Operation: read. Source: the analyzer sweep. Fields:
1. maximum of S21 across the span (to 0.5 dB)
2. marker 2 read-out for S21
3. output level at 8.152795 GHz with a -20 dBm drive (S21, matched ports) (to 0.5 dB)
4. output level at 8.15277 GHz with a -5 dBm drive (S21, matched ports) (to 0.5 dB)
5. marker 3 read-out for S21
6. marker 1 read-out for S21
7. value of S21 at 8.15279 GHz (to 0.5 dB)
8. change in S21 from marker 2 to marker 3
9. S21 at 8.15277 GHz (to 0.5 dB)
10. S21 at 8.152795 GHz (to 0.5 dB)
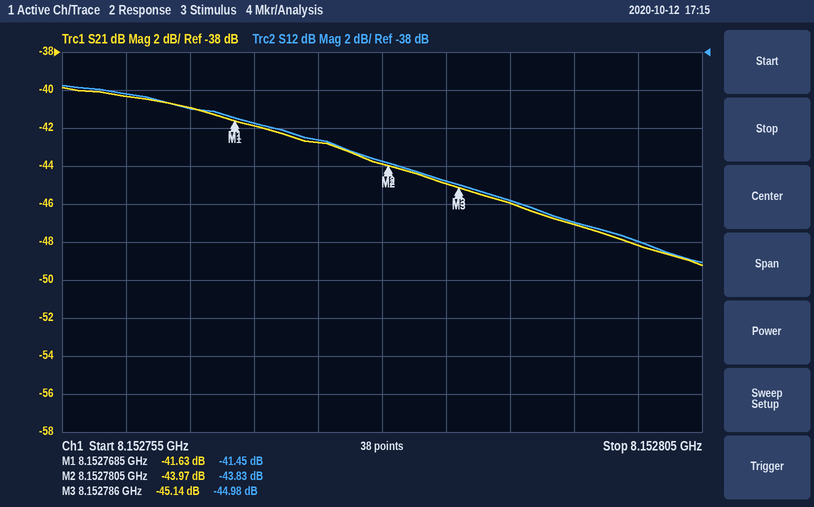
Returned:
-40.0 dB
-43.97 dB
-67.0 dBm
-47.0 dBm
-45.14 dB
-41.63 dB
-46.0 dB
-1.17 dB
-42.0 dB
-47.0 dB
